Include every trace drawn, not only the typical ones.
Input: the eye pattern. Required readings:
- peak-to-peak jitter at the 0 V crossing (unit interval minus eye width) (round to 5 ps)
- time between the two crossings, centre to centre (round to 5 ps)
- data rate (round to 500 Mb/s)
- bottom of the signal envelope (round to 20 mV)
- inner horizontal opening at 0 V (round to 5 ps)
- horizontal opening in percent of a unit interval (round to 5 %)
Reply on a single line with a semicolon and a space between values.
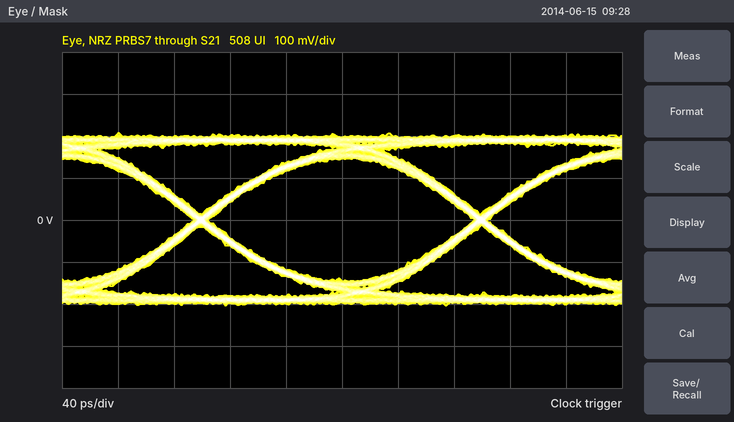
10 ps; 200 ps; 5.0 Gb/s; -200 mV; 190 ps; 95 %
